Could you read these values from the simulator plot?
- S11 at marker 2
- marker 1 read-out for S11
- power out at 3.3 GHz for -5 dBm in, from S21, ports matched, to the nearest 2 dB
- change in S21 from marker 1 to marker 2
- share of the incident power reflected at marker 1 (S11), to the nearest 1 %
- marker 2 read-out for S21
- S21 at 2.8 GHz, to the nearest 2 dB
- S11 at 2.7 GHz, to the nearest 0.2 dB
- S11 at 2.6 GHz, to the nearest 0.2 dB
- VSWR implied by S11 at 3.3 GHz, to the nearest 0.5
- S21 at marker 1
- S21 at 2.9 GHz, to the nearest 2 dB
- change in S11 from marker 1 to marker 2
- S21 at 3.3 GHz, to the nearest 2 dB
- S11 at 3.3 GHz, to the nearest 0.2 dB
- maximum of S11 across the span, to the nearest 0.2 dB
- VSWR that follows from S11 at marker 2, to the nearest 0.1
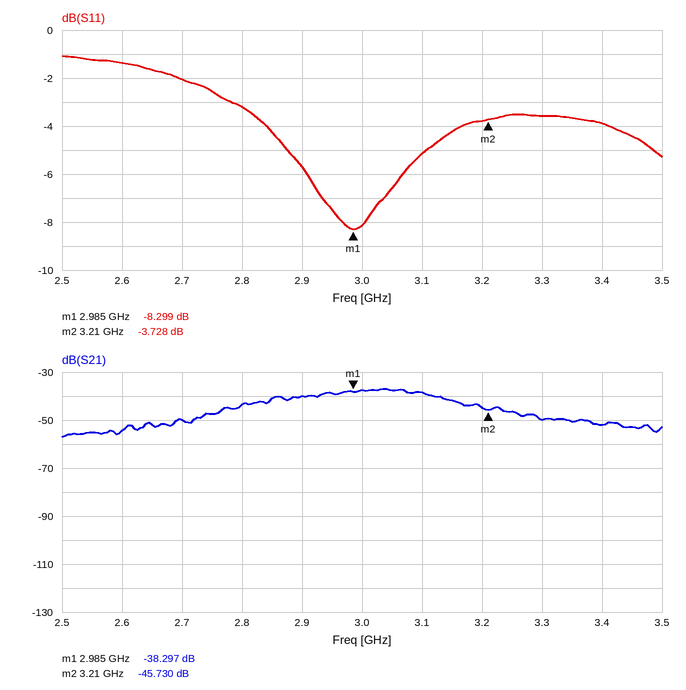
-3.728 dB
-8.299 dB
-54 dBm
-7.433 dB
15 %
-45.730 dB
-44 dB
-2.0 dB
-1.4 dB
5.0
-38.297 dB
-40 dB
4.571 dB
-50 dB
-3.6 dB
-1.0 dB
4.7
